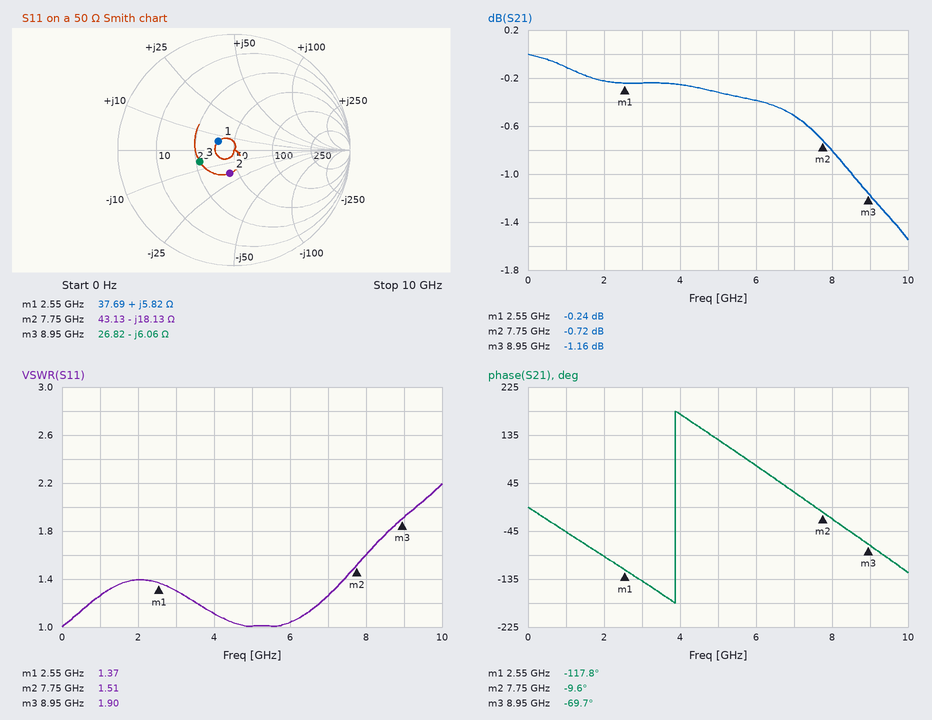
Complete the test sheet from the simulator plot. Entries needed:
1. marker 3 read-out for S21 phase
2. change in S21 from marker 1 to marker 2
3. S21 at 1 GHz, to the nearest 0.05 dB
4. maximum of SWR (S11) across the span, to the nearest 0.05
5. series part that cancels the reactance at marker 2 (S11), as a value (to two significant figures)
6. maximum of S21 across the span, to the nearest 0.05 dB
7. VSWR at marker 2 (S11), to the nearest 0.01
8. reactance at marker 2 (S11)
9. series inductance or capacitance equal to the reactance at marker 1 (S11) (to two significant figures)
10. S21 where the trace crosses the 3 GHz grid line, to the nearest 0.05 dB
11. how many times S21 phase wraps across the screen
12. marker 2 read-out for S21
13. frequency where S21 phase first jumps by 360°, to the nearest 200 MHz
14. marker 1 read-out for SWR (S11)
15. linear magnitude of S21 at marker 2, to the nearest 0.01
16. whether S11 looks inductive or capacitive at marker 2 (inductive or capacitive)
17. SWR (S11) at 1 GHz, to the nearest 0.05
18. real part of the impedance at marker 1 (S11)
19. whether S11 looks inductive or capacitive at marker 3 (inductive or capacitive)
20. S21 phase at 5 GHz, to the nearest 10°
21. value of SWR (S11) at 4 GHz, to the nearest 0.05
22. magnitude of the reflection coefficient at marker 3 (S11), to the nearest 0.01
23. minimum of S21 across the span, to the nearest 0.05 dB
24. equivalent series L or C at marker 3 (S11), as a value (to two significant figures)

-69.7°
-0.48 dB
-0.10 dB
2.20
370 pH
0.00 dB
1.51
-18.13 Ω
360 pH
-0.25 dB
1
-0.72 dB
3.8 GHz
1.37
0.92
capacitive
1.25
37.69 Ω
capacitive
130°
1.10
0.31
-1.55 dB
2.9 pF
